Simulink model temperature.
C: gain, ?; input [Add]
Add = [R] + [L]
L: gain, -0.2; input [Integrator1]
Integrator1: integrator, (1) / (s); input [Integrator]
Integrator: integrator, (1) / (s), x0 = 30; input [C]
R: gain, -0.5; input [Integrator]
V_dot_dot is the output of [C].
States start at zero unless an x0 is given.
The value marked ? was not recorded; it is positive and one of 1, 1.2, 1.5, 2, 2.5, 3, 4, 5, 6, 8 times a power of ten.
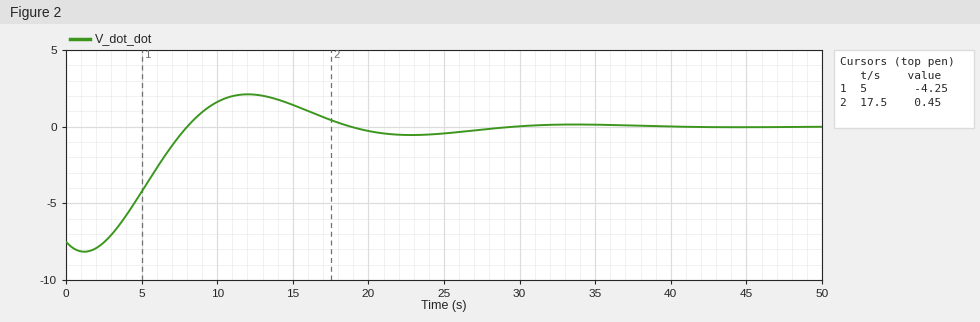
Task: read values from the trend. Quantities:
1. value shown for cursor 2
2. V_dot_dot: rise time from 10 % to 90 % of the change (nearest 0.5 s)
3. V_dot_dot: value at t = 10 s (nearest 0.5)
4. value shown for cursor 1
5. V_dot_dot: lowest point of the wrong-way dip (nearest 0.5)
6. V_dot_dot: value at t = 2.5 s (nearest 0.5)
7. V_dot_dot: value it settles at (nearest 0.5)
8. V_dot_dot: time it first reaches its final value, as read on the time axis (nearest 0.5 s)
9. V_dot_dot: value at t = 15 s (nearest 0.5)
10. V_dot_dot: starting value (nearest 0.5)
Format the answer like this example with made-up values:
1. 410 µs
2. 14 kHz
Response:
1. 0.45
2. 4.0 s
3. 1.5
4. -4.25
5. -8.0
6. -7.5
7. 0.0
8. 8.0 s
9. 1.5
10. -7.5
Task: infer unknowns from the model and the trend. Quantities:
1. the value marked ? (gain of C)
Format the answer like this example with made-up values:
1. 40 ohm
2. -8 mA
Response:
1. 0.5
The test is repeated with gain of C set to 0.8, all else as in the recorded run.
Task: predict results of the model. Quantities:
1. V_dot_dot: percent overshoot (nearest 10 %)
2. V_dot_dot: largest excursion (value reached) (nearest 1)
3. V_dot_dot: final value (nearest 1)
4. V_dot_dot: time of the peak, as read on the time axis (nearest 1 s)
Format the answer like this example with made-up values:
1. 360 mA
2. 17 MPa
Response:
1. 20 %
2. 2
3. 0
4. 9 s
